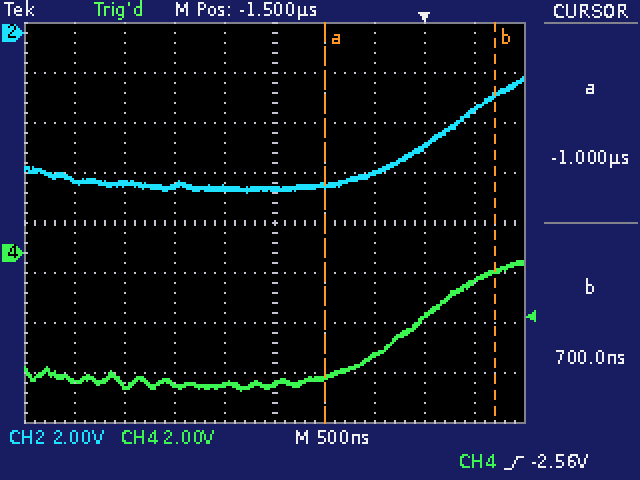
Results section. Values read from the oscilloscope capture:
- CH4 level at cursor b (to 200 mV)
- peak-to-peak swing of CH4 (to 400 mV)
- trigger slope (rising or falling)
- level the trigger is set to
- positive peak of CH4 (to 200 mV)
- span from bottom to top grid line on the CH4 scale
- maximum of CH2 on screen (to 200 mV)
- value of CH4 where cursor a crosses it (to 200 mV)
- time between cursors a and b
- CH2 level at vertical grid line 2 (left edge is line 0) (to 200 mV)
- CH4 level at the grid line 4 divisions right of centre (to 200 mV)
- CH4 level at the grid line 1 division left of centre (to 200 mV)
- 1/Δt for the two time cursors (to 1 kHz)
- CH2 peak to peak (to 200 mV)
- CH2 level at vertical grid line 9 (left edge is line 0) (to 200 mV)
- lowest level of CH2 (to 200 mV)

-800 mV
5.2 V
rising
-2.56 V
-400 mV
16 V
-1.8 V
-5.0 V
1.70 µs
-6.0 V
-1.2 V
-5.2 V
588 kHz
4.6 V
-3.0 V
-6.4 V
